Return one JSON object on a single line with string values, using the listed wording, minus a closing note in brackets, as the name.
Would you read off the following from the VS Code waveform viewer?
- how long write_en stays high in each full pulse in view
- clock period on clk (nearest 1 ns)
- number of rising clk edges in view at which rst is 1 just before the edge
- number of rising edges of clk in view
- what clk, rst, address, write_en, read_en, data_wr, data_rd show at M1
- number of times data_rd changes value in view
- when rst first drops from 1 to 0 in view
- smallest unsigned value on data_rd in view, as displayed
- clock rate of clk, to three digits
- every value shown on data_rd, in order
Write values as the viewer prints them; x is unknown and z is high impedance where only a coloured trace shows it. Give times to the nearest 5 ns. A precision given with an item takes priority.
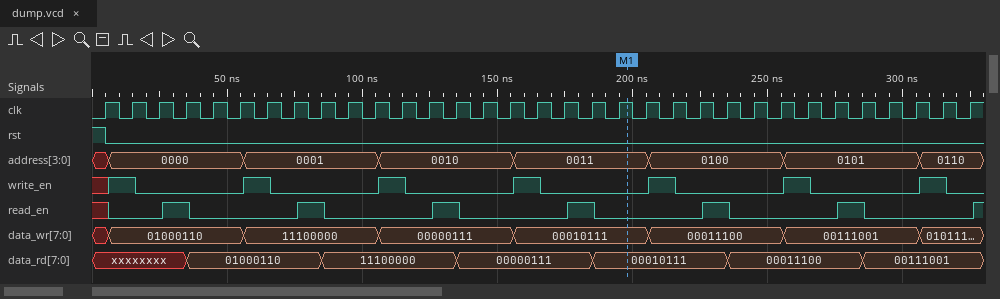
{"how long write_en stays high in each full pulse in view": "10 ns, 10 ns, 10 ns, 10 ns, 10 ns, 10 ns", "clock period on clk": "10 ns", "number of rising clk edges in view at which rst is 1 just before the edge": "1", "number of rising edges of clk in view": "33", "what clk, rst, address, write_en, read_en, data_wr, data_rd show at M1": "clk=1, rst=0, address=0011, write_en=0, read_en=0, data_wr=00010111, data_rd=00010111", "number of times data_rd changes value in view": "6", "when rst first drops from 1 to 0 in view": "5 ns", "smallest unsigned value on data_rd in view, as displayed": "00000111", "clock rate of clk, to three digits": "100 MHz", "every value shown on data_rd, in order": "xxxxxxxx, 01000110, 11100000, 00000111, 00010111, 00011100, 00111001"}
